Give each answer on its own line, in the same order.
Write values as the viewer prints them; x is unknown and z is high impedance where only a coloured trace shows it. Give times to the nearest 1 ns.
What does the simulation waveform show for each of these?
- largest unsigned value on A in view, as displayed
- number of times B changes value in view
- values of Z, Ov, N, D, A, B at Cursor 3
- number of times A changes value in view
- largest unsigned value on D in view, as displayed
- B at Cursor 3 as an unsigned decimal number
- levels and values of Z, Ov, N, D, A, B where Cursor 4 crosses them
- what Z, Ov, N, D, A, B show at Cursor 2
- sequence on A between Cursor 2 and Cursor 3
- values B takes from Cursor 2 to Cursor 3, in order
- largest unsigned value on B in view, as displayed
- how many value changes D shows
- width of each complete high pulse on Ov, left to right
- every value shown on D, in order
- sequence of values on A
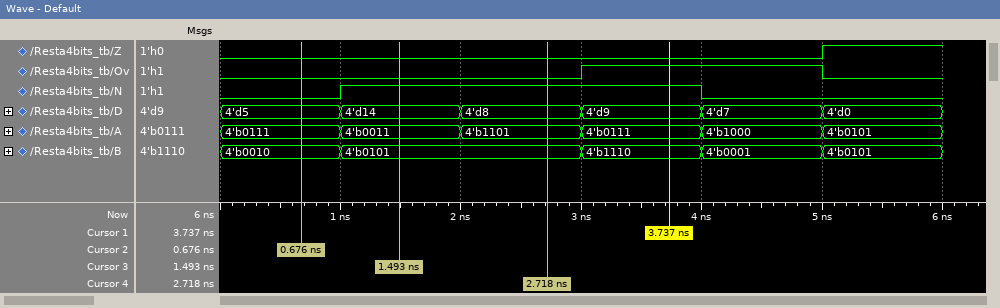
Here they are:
4'b1101
4
Z=0, Ov=0, N=1, D=4'd14, A=4'b0011, B=4'b0101
5
4'd14
5
Z=0, Ov=0, N=1, D=4'd8, A=4'b1101, B=4'b0101
Z=0, Ov=0, N=0, D=4'd5, A=4'b0111, B=4'b0010
4'b0111, 4'b0011
4'b0010, 4'b0101
4'b1110
5
2 ns
4'd5, 4'd14, 4'd8, 4'd9, 4'd7, 4'd0
4'b0111, 4'b0011, 4'b1101, 4'b0111, 4'b1000, 4'b0101
